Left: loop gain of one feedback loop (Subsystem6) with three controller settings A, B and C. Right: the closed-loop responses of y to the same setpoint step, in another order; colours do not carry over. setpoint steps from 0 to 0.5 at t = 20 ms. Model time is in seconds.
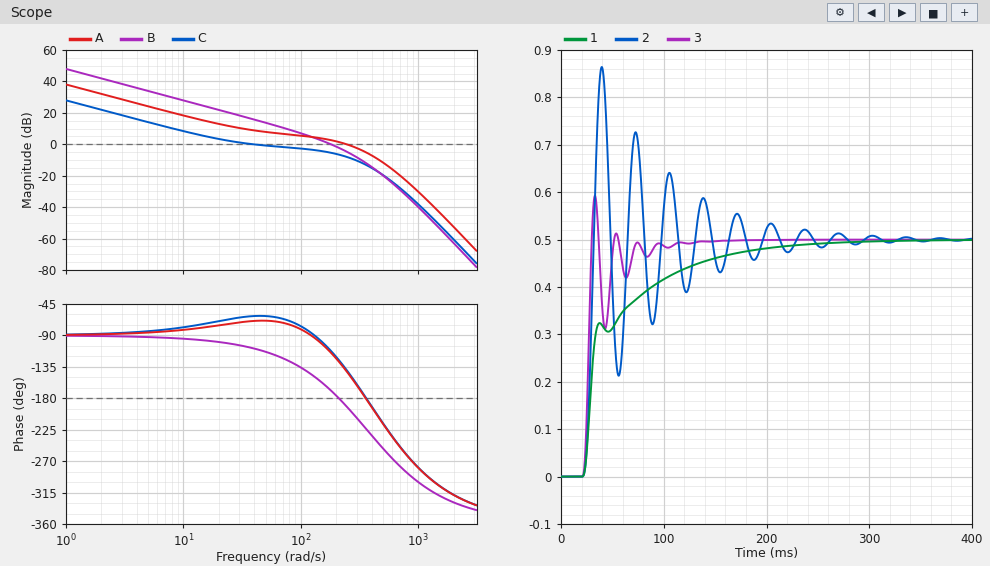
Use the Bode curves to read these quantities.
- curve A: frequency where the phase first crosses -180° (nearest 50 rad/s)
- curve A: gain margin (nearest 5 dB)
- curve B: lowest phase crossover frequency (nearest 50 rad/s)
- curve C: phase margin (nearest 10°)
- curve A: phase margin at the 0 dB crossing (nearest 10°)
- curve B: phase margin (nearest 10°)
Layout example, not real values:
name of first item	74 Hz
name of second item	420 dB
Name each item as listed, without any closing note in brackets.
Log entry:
curve A: frequency where the phase first crosses -180°	350 rad/s
curve A: gain margin	5 dB
curve B: lowest phase crossover frequency	200 rad/s
curve C: phase margin	120°
curve A: phase margin at the 0 dB crossing	40°
curve B: phase margin	10°
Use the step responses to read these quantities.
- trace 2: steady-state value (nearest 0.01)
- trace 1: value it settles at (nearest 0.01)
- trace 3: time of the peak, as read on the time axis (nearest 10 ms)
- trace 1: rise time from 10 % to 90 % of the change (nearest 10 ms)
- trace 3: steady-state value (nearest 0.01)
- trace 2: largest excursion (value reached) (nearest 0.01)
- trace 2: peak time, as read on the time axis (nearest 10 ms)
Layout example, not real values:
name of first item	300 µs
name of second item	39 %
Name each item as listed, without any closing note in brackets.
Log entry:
trace 2: steady-state value	0.50
trace 1: value it settles at	0.50
trace 3: time of the peak, as read on the time axis	30 ms
trace 1: rise time from 10 % to 90 % of the change	110 ms
trace 3: steady-state value	0.50
trace 2: largest excursion (value reached)	0.86
trace 2: peak time, as read on the time axis	40 ms
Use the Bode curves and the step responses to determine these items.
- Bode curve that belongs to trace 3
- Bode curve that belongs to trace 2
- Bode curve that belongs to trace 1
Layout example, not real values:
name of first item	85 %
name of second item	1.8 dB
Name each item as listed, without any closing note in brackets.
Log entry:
Bode curve that belongs to trace 3	A
Bode curve that belongs to trace 2	B
Bode curve that belongs to trace 1	C
